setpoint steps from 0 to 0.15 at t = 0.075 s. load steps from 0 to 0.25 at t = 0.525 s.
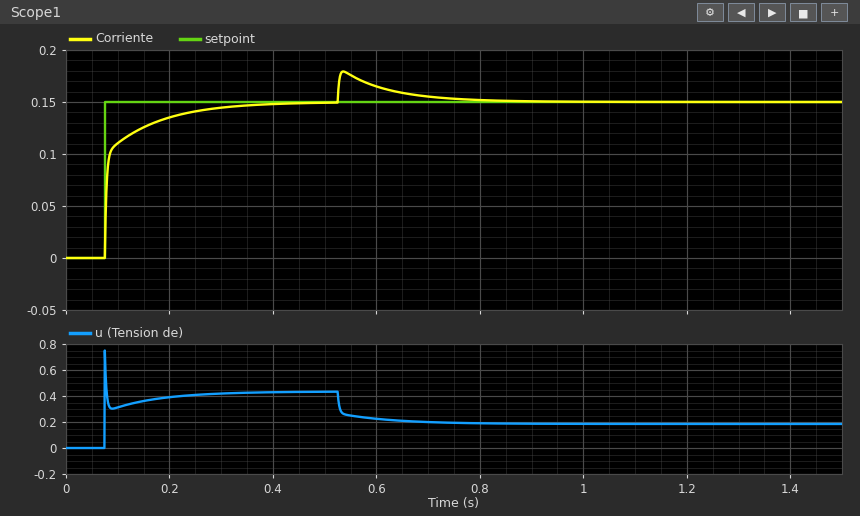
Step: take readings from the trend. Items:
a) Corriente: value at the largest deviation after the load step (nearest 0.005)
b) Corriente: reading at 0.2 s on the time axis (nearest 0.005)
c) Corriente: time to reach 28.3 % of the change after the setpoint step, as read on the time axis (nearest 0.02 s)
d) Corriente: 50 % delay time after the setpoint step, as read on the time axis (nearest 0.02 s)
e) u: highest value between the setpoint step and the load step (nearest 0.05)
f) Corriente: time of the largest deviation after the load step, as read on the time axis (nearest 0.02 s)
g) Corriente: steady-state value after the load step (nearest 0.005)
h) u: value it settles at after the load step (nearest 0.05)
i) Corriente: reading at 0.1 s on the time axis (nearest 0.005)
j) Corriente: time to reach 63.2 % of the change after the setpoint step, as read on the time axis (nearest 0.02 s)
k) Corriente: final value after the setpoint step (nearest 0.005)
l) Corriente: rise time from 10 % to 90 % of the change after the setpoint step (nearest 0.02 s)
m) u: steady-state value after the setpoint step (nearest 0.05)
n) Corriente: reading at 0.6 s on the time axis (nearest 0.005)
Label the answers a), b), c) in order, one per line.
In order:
a) 0.180
b) 0.135
c) 0.08 s
d) 0.08 s
e) 0.75
f) 0.54 s
g) 0.150
h) 0.20
i) 0.110
j) 0.08 s
k) 0.150
l) 0.12 s
m) 0.45
n) 0.165
